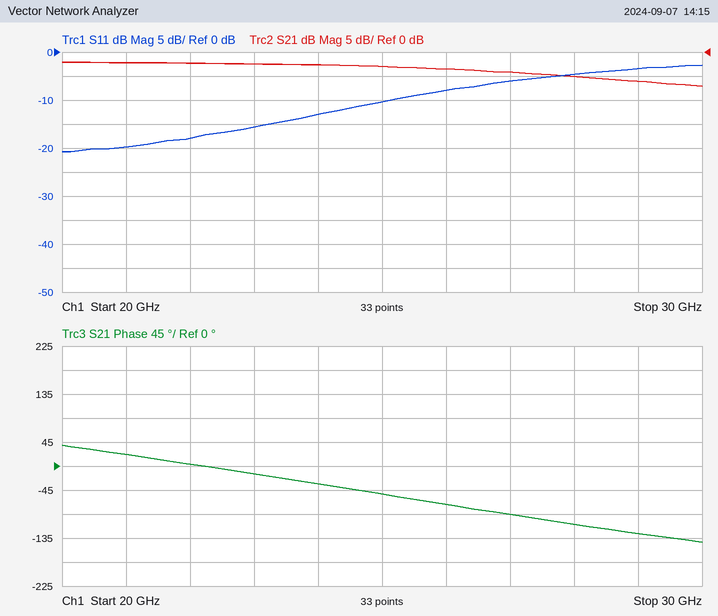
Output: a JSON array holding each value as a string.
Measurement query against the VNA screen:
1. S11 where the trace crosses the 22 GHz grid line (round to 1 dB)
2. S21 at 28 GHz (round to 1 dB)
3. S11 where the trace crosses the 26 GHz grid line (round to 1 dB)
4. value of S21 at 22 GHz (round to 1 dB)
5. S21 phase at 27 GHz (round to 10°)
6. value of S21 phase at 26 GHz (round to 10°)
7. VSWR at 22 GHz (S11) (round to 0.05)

["-18 dB", "-5 dB", "-8 dB", "-2 dB", "-90°", "-70°", "1.30"]
